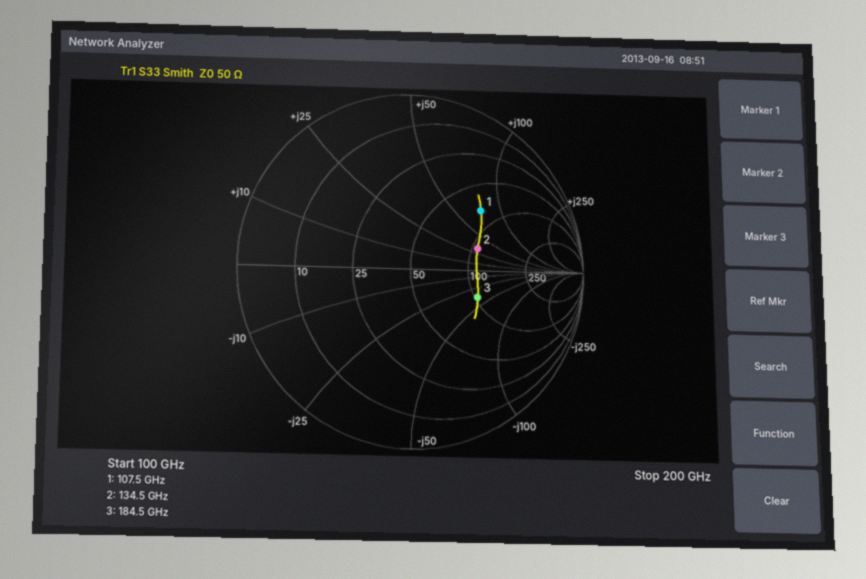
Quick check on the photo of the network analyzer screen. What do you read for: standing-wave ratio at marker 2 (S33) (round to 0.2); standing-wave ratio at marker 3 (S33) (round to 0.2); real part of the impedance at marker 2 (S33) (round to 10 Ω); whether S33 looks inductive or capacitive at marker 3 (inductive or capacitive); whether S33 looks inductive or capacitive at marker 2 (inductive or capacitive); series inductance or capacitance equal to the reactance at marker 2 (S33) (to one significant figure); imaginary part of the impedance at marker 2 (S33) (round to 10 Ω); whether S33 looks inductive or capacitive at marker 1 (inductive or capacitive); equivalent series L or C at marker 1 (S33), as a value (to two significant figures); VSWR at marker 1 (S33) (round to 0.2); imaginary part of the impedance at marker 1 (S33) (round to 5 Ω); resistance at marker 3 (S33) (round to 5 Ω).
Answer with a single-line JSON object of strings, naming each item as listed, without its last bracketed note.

{"standing-wave ratio at marker 2 (S33)": "2.4", "standing-wave ratio at marker 3 (S33)": "2.4", "real part of the impedance at marker 2 (S33)": "110 Ω", "whether S33 looks inductive or capacitive at marker 3": "capacitive", "whether S33 looks inductive or capacitive at marker 2": "inductive", "series inductance or capacitance equal to the reactance at marker 2 (S33)": "40 pH", "imaginary part of the impedance at marker 2 (S33)": "+30 Ω", "whether S33 looks inductive or capacitive at marker 1": "inductive", "equivalent series L or C at marker 1 (S33), as a value": "110 pH", "VSWR at marker 1 (S33)": "3.2", "imaginary part of the impedance at marker 1 (S33)": "+75 Ω", "resistance at marker 3 (S33)": "105 Ω"}
